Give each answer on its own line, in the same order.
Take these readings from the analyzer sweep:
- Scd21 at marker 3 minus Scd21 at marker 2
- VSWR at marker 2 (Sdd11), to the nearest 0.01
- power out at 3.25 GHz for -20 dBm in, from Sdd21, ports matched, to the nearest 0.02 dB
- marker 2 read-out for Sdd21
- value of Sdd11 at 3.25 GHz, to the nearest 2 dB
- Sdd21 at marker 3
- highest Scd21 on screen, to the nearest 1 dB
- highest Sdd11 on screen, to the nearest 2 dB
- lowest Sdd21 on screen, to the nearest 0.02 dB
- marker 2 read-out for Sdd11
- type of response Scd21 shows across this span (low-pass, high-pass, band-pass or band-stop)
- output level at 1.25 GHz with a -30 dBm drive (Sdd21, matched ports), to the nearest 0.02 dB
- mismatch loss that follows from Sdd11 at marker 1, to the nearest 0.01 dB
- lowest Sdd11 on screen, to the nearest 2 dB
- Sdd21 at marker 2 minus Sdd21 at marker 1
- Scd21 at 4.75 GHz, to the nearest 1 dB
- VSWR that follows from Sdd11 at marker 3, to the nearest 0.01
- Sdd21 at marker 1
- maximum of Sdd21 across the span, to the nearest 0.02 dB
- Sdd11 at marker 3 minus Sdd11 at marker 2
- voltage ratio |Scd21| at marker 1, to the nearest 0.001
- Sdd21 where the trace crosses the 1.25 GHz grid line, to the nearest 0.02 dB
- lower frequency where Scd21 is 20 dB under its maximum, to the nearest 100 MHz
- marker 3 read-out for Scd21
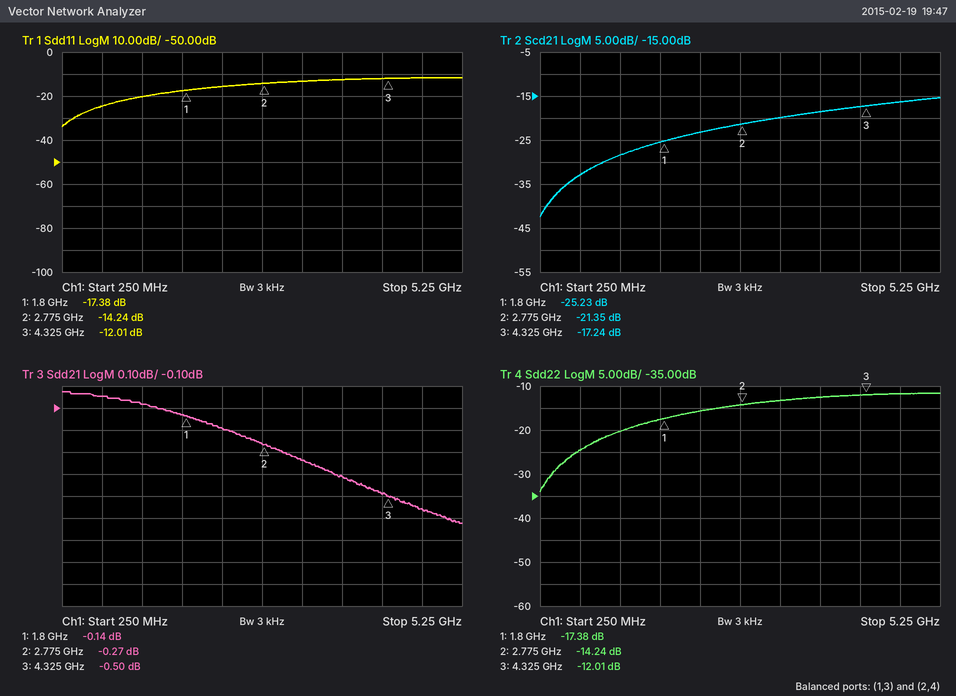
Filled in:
4.11 dB
1.48
-20.34 dBm
-0.27 dB
-14 dB
-0.50 dB
-15 dB
-12 dB
-0.62 dB
-14.24 dB
high-pass
-30.08 dBm
0.08 dB
-34 dB
-0.13 dB
-16 dB
1.67
-0.14 dB
-0.02 dB
2.23 dB
0.055
-0.08 dB
600 MHz
-17.24 dB
